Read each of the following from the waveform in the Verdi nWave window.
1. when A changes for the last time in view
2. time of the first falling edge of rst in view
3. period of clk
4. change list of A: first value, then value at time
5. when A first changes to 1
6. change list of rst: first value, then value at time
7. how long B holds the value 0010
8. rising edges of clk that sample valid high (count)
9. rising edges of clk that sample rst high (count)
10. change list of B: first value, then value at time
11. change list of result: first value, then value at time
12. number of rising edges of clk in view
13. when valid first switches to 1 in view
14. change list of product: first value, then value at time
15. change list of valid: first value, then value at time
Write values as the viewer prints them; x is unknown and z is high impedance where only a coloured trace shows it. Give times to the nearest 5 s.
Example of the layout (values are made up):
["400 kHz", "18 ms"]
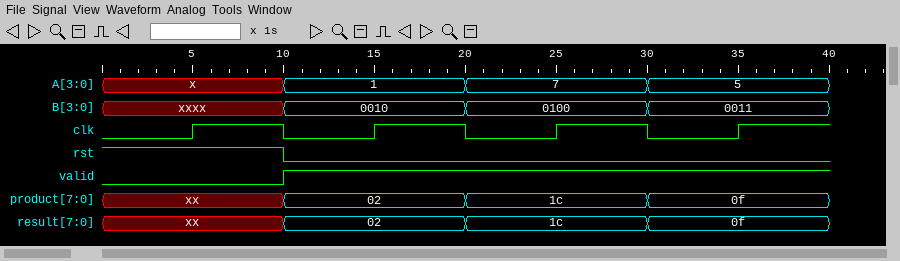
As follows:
["30 s", "10 s", "10 s", "x, 1 at 10 s, 7 at 20 s, 5 at 30 s", "10 s", "1, 0 at 10 s", "10 s", "3", "1", "xxxx, 0010 at 10 s, 0100 at 20 s, 0011 at 30 s", "xx, 02 at 10 s, 1c at 20 s, 0f at 30 s", "4", "10 s", "xx, 02 at 10 s, 1c at 20 s, 0f at 30 s", "0, 1 at 10 s"]
